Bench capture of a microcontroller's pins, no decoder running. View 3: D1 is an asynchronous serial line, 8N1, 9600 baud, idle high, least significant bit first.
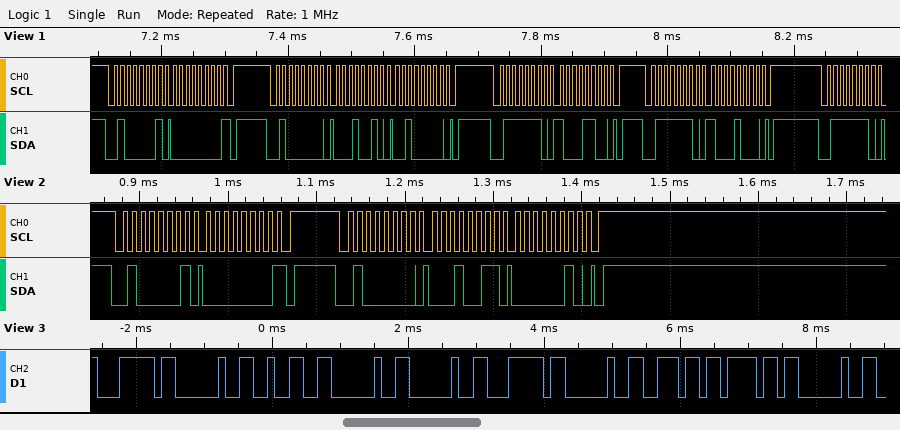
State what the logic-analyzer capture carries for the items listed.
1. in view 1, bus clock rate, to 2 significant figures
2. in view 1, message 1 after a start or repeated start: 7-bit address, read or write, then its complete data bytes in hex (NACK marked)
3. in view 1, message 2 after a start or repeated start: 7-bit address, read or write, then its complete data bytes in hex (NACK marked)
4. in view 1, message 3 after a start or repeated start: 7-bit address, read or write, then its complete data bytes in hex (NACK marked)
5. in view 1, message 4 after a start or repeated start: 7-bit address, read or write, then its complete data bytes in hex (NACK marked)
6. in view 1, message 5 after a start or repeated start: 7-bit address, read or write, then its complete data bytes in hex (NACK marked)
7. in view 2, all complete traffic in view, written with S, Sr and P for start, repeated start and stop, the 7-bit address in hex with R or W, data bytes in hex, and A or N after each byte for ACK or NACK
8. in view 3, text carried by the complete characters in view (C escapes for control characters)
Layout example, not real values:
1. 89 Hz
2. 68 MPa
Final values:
1. 100 kHz
2. 0x20 read: 00 NACK
3. 0x20 write: 12 20
4. 0x3F write: 8C
5. 0x3F write: 88
6. 0x3F write
7. S 20R A 00 N P S 20W A 13 A 02 A P
8. "| 2  | no "
